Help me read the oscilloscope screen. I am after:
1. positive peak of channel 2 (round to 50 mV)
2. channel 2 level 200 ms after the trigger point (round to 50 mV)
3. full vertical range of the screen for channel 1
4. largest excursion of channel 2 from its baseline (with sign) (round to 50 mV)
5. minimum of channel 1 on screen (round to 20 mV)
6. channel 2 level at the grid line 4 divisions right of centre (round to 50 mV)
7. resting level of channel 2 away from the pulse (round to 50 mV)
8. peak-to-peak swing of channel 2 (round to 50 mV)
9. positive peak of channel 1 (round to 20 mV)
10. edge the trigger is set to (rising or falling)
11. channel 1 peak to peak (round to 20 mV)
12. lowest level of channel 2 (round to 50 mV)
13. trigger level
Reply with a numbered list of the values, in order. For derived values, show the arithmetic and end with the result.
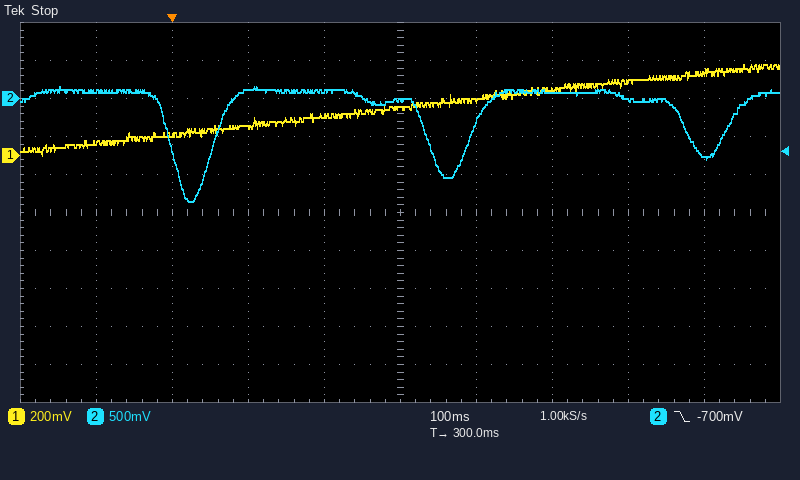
1. 150 mV
2. 100 mV
3. 2 V
4. -1.35 V − (100 mV) = -1.45 V
5. 0 mV
6. -750 mV
7. 100 mV
8. 150 mV − (-1.35 V) = 1.50 V
9. 480 mV
10. falling
11. 480 mV − (0 mV) = 480 mV
12. -1.35 V
13. -700 mV
